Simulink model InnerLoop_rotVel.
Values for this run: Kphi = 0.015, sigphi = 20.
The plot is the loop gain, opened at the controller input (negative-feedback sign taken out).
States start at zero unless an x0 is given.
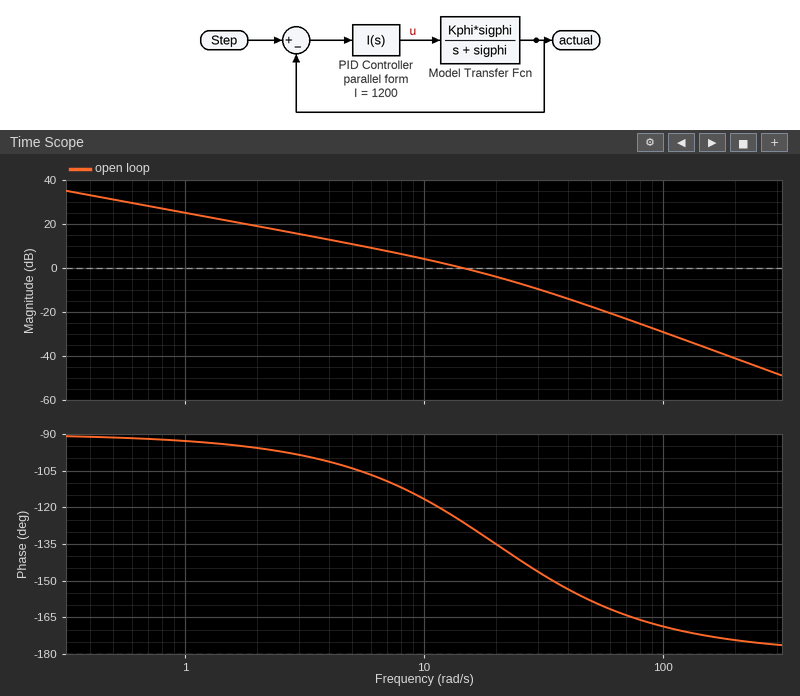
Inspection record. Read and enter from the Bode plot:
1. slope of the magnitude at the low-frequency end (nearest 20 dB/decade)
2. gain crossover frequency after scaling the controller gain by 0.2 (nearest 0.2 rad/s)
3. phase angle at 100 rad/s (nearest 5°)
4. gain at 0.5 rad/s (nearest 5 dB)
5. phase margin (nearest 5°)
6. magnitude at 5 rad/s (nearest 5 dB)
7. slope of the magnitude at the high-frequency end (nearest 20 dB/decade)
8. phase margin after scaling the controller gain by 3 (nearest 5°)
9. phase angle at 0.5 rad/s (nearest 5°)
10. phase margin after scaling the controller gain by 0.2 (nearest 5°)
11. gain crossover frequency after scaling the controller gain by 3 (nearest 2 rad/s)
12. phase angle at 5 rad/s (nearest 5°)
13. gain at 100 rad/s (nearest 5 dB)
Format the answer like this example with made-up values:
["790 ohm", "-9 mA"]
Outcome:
["-20 dB/decade", "3.6 rad/s", "-170°", "30 dB", "55°", "10 dB", "-40 dB/decade", "35°", "-90°", "80°", "30 rad/s", "-105°", "-30 dB"]
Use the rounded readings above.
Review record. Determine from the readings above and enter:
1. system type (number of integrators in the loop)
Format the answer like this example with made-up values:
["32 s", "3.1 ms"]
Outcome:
["1"]
